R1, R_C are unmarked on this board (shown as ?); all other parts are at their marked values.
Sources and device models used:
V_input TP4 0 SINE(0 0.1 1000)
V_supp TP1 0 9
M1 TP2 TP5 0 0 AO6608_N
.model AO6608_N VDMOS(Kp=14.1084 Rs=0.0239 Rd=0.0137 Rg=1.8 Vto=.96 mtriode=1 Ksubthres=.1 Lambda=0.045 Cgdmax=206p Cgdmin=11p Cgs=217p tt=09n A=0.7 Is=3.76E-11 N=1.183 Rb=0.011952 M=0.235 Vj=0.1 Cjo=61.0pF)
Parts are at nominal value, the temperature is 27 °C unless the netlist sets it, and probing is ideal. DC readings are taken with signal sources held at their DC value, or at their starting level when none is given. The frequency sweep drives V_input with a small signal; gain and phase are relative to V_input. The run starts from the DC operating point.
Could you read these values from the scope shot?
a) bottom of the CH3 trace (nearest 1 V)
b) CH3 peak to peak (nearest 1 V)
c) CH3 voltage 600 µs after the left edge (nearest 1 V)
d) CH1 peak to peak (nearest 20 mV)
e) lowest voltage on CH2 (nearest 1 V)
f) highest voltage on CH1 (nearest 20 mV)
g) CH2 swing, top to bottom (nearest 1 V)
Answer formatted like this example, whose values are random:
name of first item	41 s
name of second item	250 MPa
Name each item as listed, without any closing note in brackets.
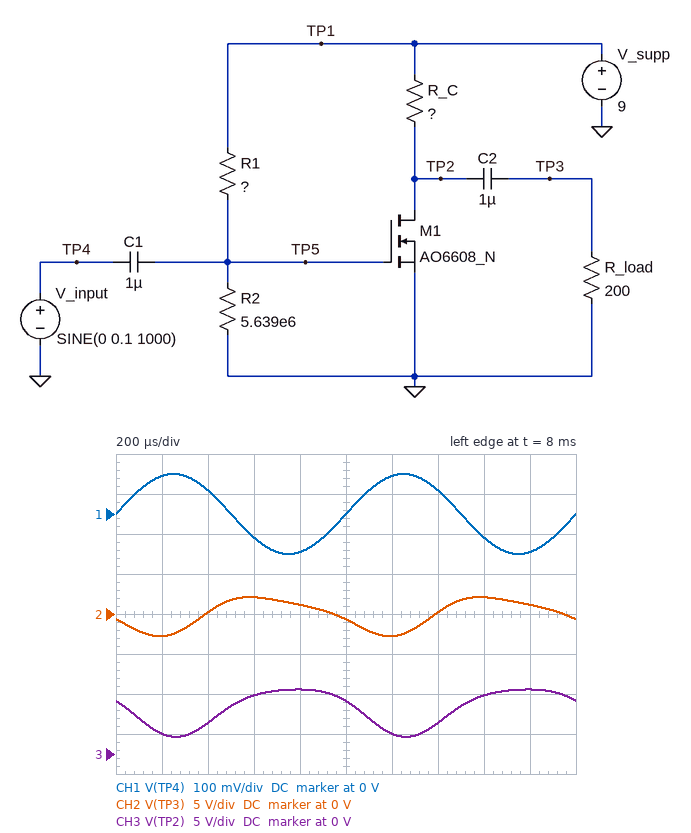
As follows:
bottom of the CH3 trace	2 V
CH3 peak to peak	6 V
CH3 voltage 600 µs after the left edge	7 V
CH1 peak to peak	200 mV
lowest voltage on CH2	-3 V
highest voltage on CH1	100 mV
CH2 swing, top to bottom	5 V
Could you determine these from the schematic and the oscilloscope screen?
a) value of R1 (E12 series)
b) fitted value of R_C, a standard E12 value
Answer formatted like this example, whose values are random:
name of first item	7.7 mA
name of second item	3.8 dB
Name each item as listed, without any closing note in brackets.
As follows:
value of R1	47 MΩ
fitted value of R_C, a standard E12 value	56 Ω
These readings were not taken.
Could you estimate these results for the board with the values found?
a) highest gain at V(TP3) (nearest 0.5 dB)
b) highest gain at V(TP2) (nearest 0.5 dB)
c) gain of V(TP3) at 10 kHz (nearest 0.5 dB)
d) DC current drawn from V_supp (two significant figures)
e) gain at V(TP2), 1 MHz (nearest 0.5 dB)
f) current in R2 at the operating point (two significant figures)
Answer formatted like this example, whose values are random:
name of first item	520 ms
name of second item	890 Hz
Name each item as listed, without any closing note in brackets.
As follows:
highest gain at V(TP3)	28.5 dB
highest gain at V(TP2)	30.5 dB
gain of V(TP3) at 10 kHz	28.5 dB
DC current drawn from V_supp	46 mA
gain at V(TP2), 1 MHz	28.5 dB
current in R2 at the operating point	170 nA
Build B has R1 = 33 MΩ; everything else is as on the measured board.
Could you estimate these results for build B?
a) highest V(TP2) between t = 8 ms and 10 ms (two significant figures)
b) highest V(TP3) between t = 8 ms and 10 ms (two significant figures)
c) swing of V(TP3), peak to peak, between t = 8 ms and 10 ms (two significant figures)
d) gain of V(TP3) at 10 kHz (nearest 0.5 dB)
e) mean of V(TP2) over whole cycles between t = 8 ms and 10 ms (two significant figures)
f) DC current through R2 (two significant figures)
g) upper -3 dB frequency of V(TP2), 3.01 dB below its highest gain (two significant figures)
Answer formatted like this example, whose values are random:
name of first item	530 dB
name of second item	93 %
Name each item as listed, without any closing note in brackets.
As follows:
highest V(TP2) between t = 8 ms and 10 ms	54 mV
highest V(TP3) between t = 8 ms and 10 ms	9.9 mV
swing of V(TP3), peak to peak, between t = 8 ms and 10 ms	18 mV
gain of V(TP3) at 10 kHz	-20.0 dB
mean of V(TP2) over whole cycles between t = 8 ms and 10 ms	41 mV
DC current through R2	230 nA
upper -3 dB frequency of V(TP2), 3.01 dB below its highest gain	450 MHz
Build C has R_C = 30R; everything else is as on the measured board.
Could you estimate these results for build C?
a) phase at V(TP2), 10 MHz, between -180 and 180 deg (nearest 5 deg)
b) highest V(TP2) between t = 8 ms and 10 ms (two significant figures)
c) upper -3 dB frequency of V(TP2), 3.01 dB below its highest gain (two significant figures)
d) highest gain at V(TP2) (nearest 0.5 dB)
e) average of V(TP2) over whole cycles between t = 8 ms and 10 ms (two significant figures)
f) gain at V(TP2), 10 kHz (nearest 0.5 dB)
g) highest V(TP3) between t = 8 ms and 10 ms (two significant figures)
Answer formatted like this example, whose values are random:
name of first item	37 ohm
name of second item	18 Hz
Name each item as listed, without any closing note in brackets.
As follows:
phase at V(TP2), 10 MHz, between -180 and 180 deg	170 deg
highest V(TP2) between t = 8 ms and 10 ms	8.6 V
upper -3 dB frequency of V(TP2), 3.01 dB below its highest gain	51 MHz
highest gain at V(TP2)	25.5 dB
average of V(TP2) over whole cycles between t = 8 ms and 10 ms	7.1 V
gain at V(TP2), 10 kHz	24.5 dB
highest V(TP3) between t = 8 ms and 10 ms	1.4 V
